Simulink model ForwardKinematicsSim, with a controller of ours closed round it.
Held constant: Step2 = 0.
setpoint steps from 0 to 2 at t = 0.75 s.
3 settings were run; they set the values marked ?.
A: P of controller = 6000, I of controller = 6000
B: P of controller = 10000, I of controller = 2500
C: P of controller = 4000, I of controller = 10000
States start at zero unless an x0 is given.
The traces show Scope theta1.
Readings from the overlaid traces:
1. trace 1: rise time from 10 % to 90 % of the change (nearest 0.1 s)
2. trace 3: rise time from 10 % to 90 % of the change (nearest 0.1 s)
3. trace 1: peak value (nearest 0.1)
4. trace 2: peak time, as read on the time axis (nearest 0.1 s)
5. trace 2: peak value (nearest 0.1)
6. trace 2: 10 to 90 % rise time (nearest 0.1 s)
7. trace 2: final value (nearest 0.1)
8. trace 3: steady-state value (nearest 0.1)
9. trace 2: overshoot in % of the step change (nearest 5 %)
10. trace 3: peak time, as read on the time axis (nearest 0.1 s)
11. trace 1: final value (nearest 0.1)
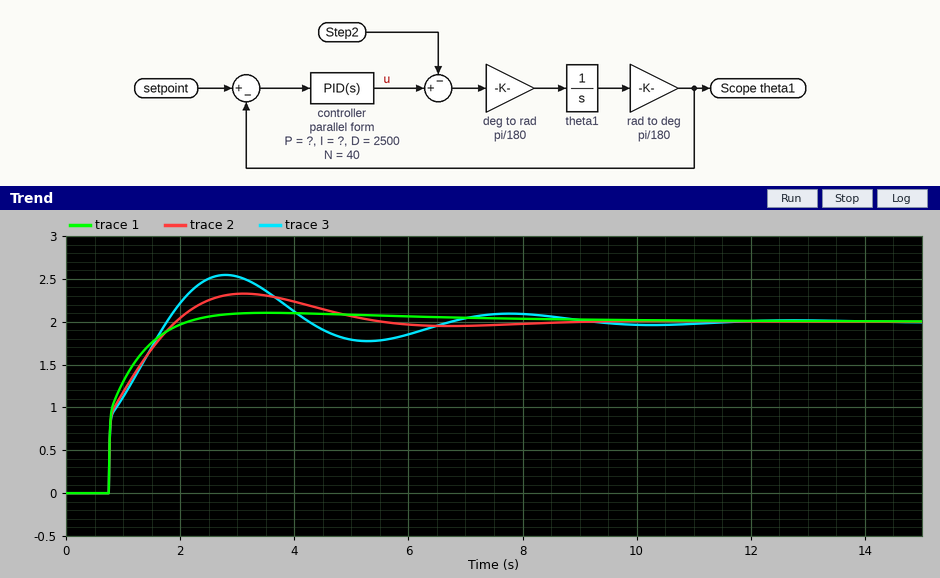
0.8 s
0.8 s
2.1
3.1 s
2.3
0.9 s
2.0
2.0
15 %
2.8 s
2.0
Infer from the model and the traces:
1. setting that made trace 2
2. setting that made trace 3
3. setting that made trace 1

A
C
B
